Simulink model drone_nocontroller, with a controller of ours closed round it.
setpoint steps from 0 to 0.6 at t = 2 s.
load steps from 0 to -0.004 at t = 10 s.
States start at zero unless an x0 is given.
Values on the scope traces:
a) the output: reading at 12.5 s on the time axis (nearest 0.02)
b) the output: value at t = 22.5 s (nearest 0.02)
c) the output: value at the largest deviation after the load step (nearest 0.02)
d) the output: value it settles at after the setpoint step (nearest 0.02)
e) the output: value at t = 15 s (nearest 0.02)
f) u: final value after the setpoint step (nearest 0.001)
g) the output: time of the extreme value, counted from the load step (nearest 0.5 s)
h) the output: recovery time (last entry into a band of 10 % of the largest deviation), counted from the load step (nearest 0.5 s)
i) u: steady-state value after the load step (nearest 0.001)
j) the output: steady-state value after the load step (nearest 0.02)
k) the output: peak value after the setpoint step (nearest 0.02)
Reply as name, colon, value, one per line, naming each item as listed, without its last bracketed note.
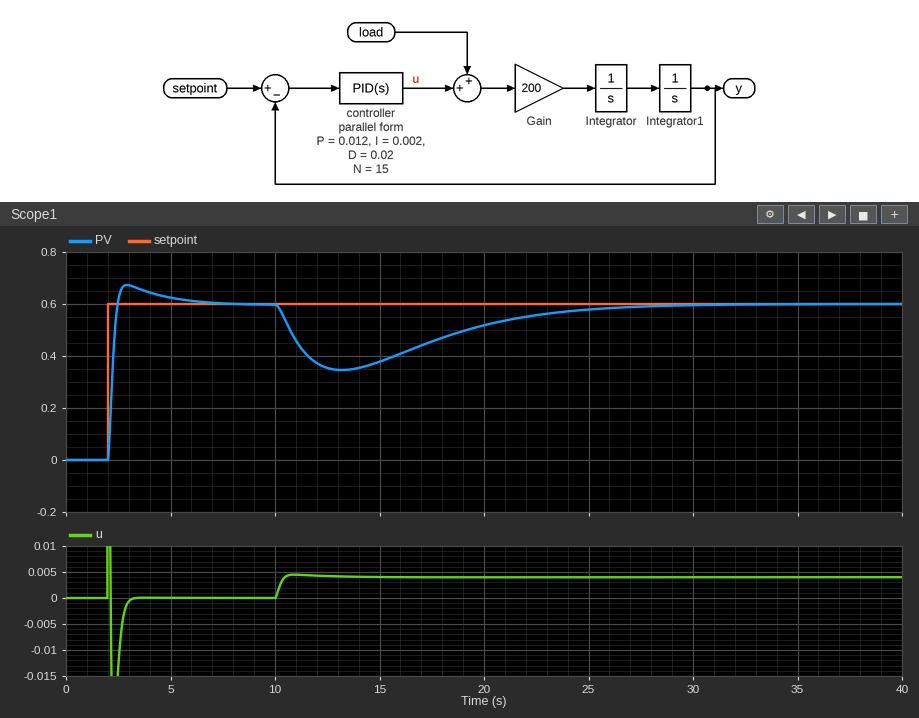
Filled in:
the output: reading at 12.5 s on the time axis: 0.36
the output: value at t = 22.5 s: 0.56
the output: value at the largest deviation after the load step: 0.34
the output: value it settles at after the setpoint step: 0.60
the output: value at t = 15 s: 0.38
u: final value after the setpoint step: 0.000
the output: time of the extreme value, counted from the load step: 3.0 s
the output: recovery time (last entry into a band of 10 % of the largest deviation), counted from the load step: 14.5 s
u: steady-state value after the load step: 0.004
the output: steady-state value after the load step: 0.60
the output: peak value after the setpoint step: 0.68
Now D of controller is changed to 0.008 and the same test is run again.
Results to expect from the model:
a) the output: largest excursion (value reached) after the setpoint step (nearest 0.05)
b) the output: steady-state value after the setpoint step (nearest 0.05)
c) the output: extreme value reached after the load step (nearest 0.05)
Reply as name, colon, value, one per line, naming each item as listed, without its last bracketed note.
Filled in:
the output: largest excursion (value reached) after the setpoint step: 0.80
the output: steady-state value after the setpoint step: 0.60
the output: extreme value reached after the load step: 0.25
